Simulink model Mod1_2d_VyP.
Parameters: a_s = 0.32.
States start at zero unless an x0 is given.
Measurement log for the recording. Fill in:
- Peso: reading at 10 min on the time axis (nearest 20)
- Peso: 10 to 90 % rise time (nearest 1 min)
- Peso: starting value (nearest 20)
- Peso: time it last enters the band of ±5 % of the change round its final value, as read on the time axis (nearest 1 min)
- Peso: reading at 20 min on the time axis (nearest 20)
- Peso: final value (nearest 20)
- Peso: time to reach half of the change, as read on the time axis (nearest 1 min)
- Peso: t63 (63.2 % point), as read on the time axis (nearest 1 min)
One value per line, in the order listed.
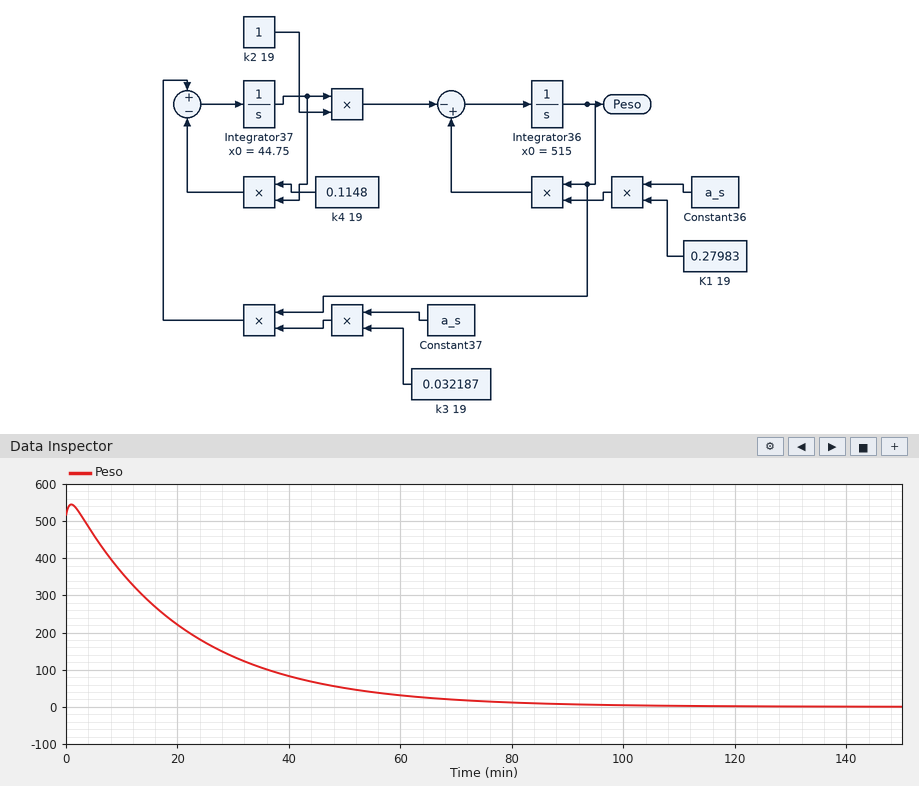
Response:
360
45 min
520
64 min
220
0
17 min
23 min
